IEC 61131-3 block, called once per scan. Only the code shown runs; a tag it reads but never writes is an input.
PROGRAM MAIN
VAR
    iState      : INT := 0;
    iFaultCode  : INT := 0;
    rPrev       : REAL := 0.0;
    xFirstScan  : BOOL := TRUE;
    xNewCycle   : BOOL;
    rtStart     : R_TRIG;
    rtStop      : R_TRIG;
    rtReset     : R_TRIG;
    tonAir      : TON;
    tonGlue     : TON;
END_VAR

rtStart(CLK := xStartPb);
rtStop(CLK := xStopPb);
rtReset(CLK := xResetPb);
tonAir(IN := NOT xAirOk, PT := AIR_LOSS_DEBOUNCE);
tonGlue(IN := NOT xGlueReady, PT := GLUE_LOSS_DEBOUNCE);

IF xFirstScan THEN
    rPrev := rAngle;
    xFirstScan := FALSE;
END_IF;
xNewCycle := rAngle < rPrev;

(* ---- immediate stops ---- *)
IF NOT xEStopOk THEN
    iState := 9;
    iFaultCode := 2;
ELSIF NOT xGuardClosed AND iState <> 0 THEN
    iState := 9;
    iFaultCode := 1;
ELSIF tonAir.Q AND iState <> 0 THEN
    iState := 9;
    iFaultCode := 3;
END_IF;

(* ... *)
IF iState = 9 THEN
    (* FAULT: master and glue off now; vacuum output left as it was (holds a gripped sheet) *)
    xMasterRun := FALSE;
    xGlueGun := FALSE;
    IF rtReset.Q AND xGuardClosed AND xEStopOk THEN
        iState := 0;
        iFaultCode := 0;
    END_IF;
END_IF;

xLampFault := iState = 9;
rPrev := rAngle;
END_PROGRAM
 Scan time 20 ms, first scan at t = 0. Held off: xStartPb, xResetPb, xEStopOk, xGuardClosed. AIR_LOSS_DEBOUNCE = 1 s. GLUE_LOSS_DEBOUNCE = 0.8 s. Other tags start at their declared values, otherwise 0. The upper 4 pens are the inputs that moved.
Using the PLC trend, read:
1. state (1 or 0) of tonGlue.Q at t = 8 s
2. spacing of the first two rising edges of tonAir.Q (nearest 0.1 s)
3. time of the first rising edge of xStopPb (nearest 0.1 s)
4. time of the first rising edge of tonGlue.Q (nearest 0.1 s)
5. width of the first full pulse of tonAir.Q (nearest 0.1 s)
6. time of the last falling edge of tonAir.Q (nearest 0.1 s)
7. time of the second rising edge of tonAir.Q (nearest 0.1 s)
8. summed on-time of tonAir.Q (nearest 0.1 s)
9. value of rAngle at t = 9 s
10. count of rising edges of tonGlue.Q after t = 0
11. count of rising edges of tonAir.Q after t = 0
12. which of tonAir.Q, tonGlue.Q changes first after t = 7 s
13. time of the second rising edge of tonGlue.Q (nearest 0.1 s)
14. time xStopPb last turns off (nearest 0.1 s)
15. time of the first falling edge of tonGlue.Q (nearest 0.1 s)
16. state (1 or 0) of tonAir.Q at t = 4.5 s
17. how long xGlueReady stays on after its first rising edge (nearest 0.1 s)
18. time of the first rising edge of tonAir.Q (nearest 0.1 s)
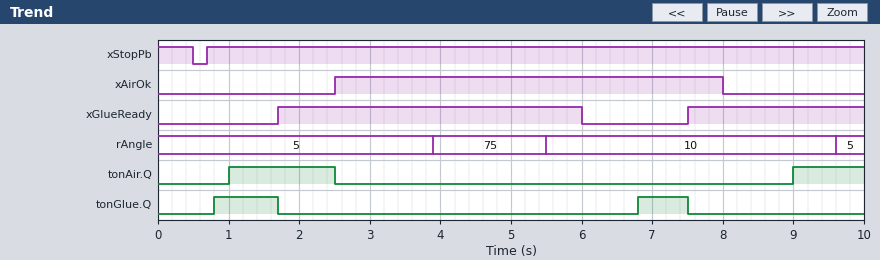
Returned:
0
8.0 s
0.7 s
0.8 s
1.5 s
2.5 s
9.0 s
2.5 s
10
2
2
tonGlue.Q
6.8 s
0.5 s
1.7 s
0
4.3 s
1.0 s
